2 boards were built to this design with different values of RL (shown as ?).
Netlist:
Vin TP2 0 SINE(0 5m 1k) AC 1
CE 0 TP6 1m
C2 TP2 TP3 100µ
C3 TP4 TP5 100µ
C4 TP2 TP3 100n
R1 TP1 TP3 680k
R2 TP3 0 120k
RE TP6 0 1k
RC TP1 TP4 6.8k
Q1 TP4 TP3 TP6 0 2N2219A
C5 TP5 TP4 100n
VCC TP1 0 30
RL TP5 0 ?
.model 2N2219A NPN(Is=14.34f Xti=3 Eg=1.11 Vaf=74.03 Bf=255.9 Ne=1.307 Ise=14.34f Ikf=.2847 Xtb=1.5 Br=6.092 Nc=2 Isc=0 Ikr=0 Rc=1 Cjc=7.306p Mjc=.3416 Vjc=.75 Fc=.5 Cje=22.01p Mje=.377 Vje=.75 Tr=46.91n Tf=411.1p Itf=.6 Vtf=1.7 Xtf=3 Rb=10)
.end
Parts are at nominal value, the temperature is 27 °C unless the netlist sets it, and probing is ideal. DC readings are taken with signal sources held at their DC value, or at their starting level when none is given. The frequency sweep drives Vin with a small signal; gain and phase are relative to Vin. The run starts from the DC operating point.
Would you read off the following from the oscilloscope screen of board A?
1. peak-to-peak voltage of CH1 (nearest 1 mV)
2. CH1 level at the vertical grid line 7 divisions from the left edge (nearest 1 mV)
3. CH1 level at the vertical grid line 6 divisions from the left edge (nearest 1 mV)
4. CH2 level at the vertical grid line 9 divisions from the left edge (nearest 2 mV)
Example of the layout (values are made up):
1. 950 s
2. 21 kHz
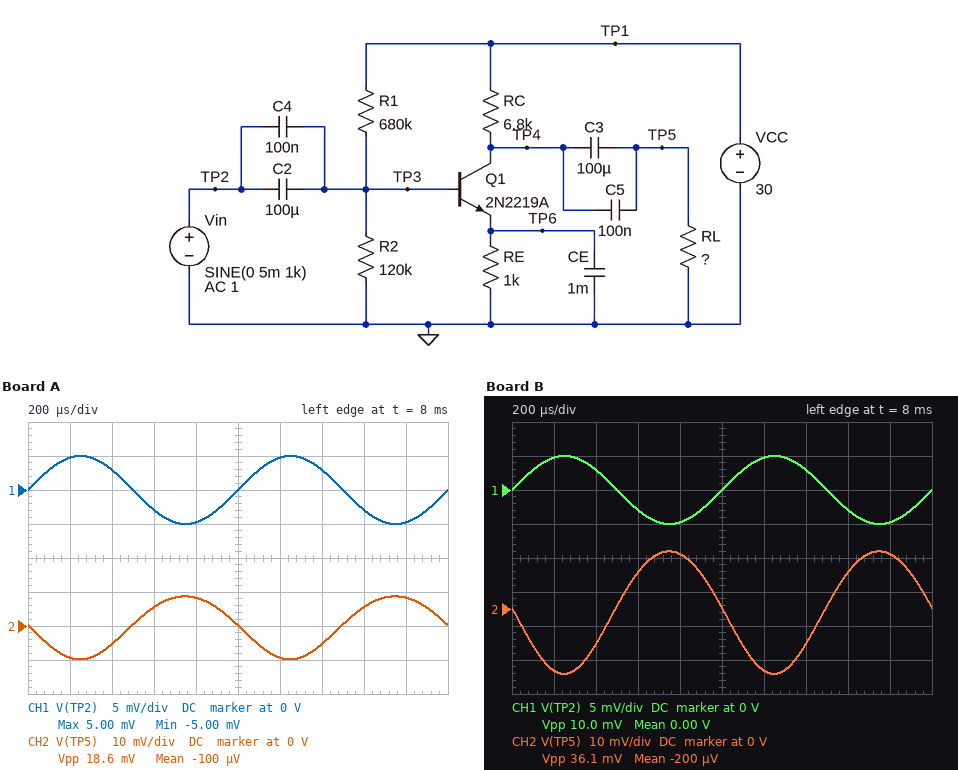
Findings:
1. 10 mV
2. 3 mV
3. 5 mV
4. 8 mV
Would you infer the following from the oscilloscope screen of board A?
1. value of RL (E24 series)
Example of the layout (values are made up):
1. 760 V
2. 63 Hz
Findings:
1. 20 Ω
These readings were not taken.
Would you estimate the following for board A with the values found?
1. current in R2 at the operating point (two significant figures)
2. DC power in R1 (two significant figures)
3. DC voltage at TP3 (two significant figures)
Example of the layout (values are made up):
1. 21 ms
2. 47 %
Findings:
1. 26 µA
2. 1.1 mW
3. 3.1 V
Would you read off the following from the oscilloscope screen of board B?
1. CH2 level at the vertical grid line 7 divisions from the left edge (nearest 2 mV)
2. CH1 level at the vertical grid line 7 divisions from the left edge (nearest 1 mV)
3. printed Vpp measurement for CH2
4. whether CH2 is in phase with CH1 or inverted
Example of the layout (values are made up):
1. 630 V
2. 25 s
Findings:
1. -10 mV
2. 3 mV
3. 36.1 mV
4. inverted
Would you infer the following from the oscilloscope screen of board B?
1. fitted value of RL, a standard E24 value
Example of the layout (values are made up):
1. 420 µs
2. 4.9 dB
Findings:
1. 39 Ω
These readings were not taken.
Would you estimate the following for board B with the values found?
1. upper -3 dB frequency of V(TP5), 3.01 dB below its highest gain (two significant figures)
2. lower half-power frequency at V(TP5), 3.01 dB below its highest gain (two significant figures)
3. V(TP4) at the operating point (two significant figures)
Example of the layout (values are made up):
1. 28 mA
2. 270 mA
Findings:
1. 170 MHz
2. 16 Hz
3. 13 V
